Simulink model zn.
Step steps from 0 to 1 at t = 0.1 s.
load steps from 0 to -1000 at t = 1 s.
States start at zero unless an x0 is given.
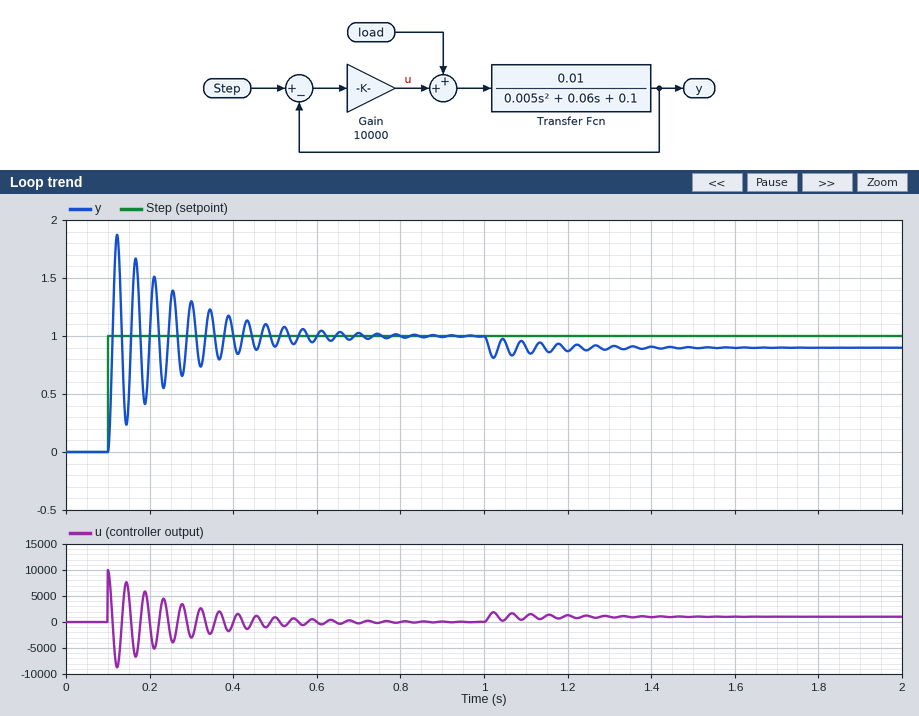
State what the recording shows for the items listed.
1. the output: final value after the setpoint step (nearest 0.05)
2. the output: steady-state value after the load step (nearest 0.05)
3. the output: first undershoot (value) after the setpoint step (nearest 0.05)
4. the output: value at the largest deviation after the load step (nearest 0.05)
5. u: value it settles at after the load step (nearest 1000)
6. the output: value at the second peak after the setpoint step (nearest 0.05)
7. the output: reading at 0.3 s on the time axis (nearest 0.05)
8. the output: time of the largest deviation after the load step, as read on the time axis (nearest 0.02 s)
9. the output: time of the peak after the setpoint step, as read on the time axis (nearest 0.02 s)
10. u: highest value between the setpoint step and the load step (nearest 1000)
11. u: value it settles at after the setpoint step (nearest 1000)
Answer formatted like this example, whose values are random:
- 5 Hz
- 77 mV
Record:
- 1.00
- 0.90
- 0.25
- 0.80
- 1000
- 1.65
- 1.30
- 1.02 s
- 0.12 s
- 10000
- 0
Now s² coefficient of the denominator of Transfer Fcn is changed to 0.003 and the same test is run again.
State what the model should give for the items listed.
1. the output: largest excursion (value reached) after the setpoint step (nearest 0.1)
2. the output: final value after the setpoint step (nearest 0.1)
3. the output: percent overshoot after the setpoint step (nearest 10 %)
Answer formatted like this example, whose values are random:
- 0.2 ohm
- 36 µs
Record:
- 1.8
- 1.0
- 80 %
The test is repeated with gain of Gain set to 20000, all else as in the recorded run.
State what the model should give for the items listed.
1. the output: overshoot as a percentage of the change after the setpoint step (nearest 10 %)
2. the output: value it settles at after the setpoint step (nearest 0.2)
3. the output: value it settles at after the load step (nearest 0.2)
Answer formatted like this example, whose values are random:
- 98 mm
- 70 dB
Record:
- 90 %
- 1.0
- 1.0
